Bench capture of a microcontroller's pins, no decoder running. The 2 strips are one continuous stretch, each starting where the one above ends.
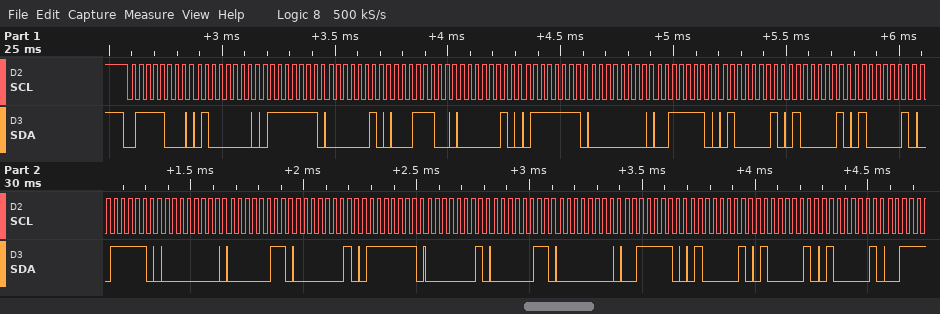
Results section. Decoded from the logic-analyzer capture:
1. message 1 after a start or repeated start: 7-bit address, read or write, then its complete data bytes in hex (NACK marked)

0x3C write: 40 7F 02 1C 02 7F 00 3E 41 41 41 3E 00 03 01 7F 01 03 00 3E 41 41 41
